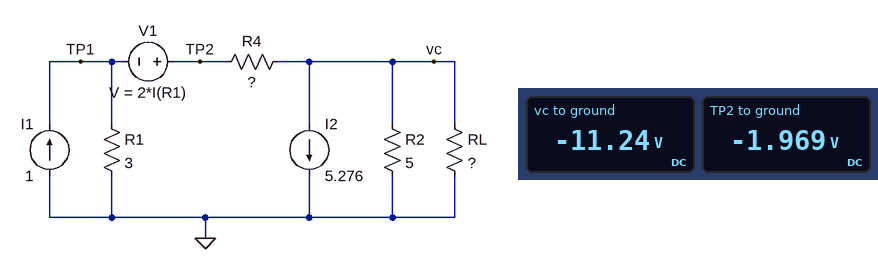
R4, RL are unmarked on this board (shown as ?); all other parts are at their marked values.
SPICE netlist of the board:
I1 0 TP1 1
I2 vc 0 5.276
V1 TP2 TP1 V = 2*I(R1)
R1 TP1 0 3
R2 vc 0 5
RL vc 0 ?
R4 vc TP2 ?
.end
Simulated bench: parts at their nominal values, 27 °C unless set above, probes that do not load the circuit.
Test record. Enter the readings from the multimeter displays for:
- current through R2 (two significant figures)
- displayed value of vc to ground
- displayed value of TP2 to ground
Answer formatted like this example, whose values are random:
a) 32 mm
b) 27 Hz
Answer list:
a) 2.2 A
b) -11.24 V
c) -1.969 V
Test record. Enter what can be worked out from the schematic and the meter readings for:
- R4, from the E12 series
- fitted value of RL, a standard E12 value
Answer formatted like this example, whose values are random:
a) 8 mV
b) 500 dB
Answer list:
a) 5.6 Ω
b) 8.2 Ω
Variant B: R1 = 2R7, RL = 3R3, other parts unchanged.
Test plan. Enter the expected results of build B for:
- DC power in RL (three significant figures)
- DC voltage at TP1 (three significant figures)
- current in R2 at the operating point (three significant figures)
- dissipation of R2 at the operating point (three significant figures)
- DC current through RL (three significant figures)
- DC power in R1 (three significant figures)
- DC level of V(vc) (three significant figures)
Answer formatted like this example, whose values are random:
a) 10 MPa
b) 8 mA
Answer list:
a) 19.1 W
b) -761 mV
c) 1.59 A
d) 12.6 W
e) 2.41 A
f) 215 mW
g) -7.94 V
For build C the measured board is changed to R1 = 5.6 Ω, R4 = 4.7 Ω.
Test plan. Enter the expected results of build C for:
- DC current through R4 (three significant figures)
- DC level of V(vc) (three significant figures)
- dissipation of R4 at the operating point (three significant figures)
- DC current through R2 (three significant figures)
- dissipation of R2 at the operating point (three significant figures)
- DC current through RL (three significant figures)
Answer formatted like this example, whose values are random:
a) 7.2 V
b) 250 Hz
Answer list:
a) 1.64 A
b) -11.3 V
c) 12.6 W
d) 2.26 A
e) 25.5 W
f) 1.38 A
